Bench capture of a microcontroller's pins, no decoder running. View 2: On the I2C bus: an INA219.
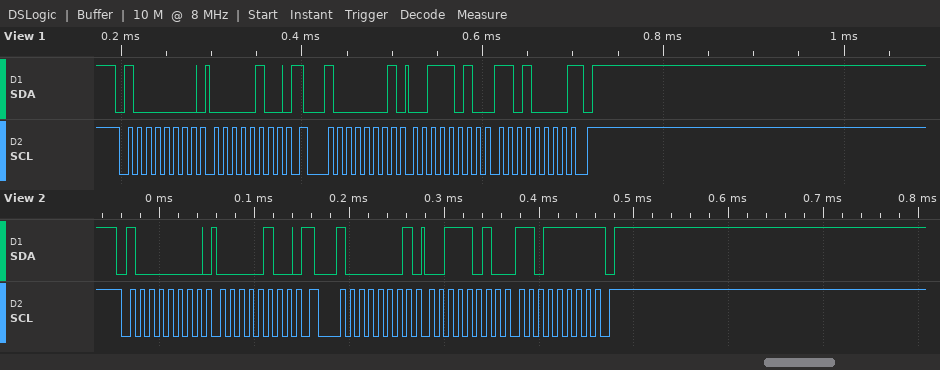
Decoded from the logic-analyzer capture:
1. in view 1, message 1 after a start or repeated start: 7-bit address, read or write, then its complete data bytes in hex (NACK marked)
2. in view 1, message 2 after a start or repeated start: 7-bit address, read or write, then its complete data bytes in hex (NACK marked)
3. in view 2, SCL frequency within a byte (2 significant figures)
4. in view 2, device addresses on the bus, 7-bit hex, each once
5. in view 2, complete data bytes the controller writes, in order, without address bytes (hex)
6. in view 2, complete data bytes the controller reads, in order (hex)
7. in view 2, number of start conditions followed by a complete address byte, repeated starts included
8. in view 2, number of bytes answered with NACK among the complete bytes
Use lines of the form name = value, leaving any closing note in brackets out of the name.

in view 1, message 1 after a start or repeated start: 7-bit address, read or write, then its complete data bytes in hex = 0x40 write: 04
in view 1, message 2 after a start or repeated start: 7-bit address, read or write, then its complete data bytes in hex = 0x40 read: 3A D0 NACK
in view 2, SCL frequency within a byte = 100 kHz
in view 2, device addresses on the bus, 7-bit hex, each once = 0x40
in view 2, complete data bytes the controller writes, in order, without address bytes = 04
in view 2, complete data bytes the controller reads, in order = 3A DF
in view 2, number of start conditions followed by a complete address byte, repeated starts included = 2
in view 2, number of bytes answered with NACK among the complete bytes = 1
